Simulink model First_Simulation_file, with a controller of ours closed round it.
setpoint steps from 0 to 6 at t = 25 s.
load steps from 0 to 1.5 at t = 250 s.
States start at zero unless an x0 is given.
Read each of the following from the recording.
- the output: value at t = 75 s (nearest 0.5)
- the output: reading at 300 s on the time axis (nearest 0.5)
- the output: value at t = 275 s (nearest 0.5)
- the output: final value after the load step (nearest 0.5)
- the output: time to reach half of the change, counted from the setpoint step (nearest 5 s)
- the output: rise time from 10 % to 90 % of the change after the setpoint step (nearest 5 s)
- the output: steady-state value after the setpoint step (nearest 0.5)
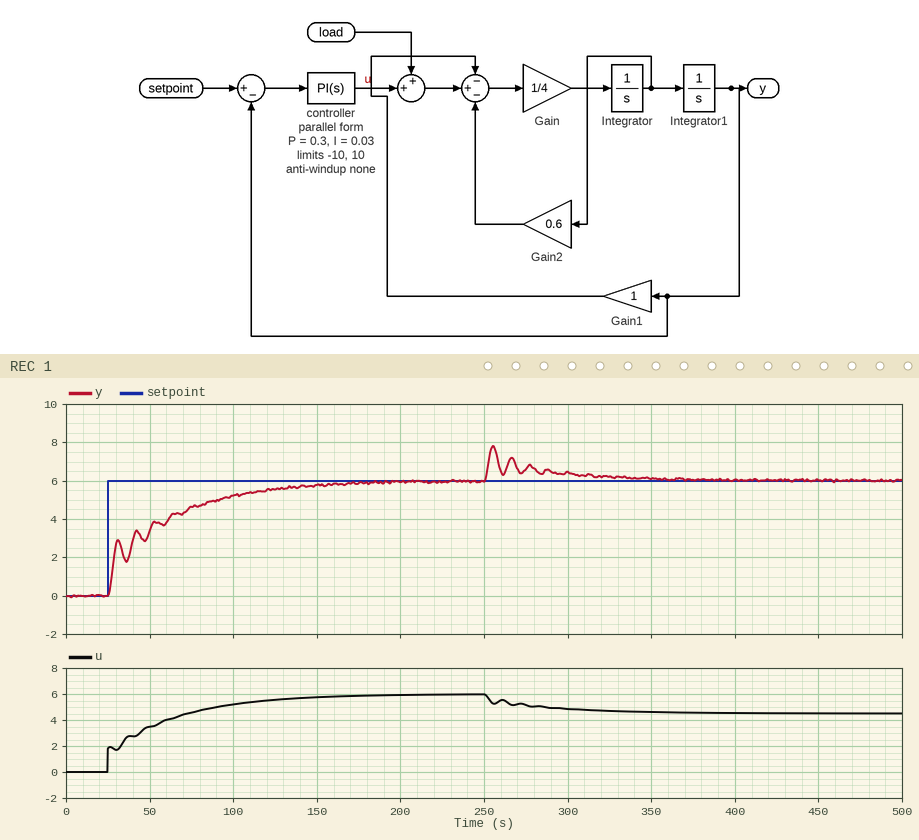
4.5
6.5
6.5
6.0
15 s
85 s
6.0
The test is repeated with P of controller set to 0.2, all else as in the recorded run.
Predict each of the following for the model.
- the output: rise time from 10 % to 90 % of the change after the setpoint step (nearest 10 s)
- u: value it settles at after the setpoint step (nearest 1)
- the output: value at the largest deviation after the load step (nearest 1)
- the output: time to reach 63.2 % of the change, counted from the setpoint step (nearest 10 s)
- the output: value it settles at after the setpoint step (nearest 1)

80 s
6
8
30 s
6
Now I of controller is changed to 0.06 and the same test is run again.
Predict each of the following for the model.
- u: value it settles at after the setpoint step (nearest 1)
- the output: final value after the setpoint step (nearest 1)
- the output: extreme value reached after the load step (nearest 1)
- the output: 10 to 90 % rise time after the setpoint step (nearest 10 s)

6
6
8
40 s
